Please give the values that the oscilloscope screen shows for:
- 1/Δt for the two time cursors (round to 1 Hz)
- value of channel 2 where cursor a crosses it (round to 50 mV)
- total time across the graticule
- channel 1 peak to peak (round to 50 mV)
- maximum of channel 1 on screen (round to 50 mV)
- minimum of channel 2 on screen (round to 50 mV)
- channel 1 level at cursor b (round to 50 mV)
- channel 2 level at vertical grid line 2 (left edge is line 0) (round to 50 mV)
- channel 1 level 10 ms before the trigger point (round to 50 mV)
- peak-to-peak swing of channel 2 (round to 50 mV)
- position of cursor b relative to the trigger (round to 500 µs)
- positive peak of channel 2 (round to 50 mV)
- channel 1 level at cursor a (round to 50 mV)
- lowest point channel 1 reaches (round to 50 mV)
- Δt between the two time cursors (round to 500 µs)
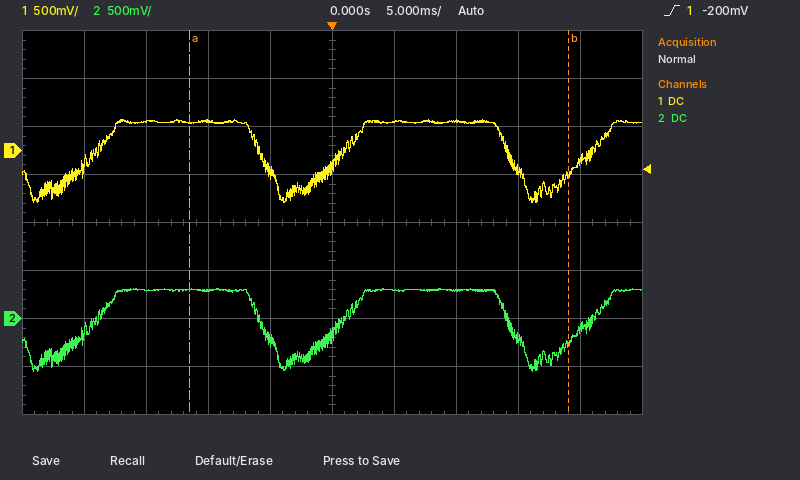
33 Hz
300 mV
50 ms
850 mV
300 mV
-550 mV
-250 mV
300 mV
300 mV
850 mV
+19.0 ms
300 mV
300 mV
-550 mV
30.5 ms
